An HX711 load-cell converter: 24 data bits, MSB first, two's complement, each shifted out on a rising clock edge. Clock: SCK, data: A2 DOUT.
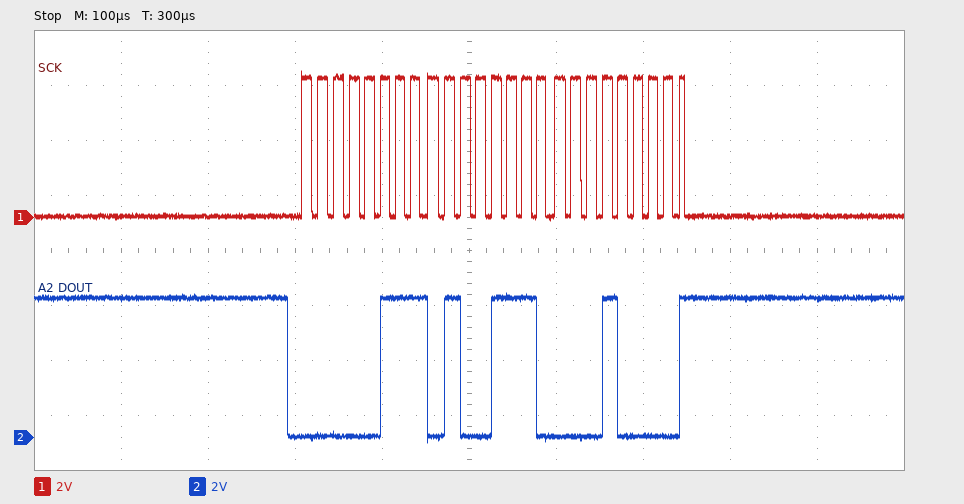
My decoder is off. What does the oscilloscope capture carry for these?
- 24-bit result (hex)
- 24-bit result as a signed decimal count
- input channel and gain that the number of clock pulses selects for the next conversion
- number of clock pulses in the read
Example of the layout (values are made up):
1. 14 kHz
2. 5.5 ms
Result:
1. 0x074E10
2. 478736
3. channel A, gain 128
4. 25
